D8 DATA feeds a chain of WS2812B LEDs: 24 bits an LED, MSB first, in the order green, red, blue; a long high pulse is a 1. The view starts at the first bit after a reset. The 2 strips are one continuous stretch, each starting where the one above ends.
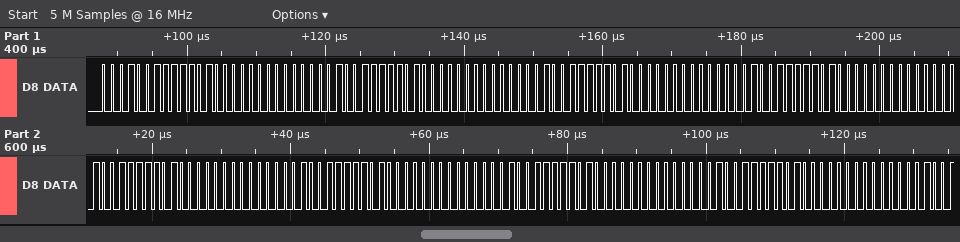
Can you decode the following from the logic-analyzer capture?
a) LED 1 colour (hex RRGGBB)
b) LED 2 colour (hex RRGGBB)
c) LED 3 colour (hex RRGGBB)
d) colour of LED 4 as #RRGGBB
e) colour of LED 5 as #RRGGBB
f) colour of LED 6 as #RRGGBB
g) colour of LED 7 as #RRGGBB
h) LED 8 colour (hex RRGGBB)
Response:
#E81300
#E81300
#E81300
#E81300
#E81300
#E81300
#E81300
#E81300
